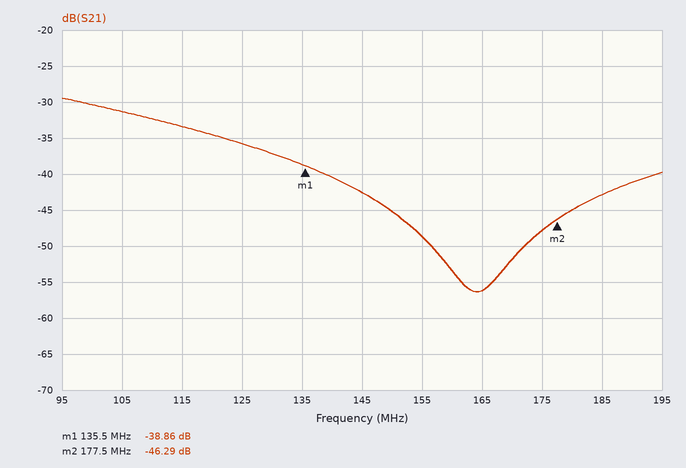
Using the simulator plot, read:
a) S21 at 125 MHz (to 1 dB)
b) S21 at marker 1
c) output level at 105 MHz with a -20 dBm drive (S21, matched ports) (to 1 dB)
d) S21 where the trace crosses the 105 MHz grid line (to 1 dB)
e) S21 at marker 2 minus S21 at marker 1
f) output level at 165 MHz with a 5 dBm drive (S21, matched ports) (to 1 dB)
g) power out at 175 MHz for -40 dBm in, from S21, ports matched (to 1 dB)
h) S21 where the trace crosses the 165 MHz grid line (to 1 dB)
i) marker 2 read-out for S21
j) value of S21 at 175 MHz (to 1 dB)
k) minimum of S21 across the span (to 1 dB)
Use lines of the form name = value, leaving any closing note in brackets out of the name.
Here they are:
S21 at 125 MHz = -36 dB
S21 at marker 1 = -38.86 dB
output level at 105 MHz with a -20 dBm drive (S21, matched ports) = -51 dBm
S21 where the trace crosses the 105 MHz grid line = -31 dB
S21 at marker 2 minus S21 at marker 1 = -7.43 dB
output level at 165 MHz with a 5 dBm drive (S21, matched ports) = -51 dBm
power out at 175 MHz for -40 dBm in, from S21, ports matched = -88 dBm
S21 where the trace crosses the 165 MHz grid line = -56 dB
marker 2 read-out for S21 = -46.29 dB
value of S21 at 175 MHz = -48 dB
minimum of S21 across the span = -56 dB
